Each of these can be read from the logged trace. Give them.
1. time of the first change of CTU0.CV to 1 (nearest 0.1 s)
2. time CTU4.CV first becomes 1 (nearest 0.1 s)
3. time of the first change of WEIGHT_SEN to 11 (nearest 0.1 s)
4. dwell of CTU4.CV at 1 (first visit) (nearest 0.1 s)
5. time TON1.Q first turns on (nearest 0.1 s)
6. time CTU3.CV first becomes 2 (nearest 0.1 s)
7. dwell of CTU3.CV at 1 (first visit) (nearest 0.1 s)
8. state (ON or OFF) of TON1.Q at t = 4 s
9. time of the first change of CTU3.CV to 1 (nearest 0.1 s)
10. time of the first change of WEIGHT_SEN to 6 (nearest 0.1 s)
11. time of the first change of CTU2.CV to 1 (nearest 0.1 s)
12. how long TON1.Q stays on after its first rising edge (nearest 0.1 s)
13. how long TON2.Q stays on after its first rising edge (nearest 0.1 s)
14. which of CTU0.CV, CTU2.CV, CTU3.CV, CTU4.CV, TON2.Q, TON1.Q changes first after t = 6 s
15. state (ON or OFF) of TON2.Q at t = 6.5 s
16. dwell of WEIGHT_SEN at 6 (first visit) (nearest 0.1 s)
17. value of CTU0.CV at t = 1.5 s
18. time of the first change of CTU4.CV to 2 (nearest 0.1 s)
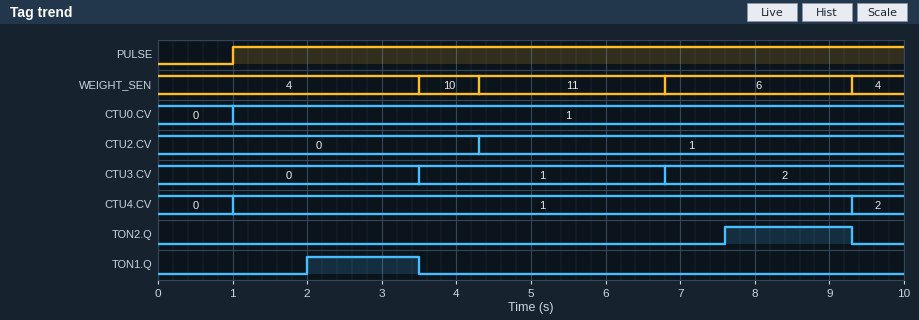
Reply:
1.0 s
1.0 s
4.3 s
8.3 s
2.0 s
6.8 s
3.3 s
OFF
3.5 s
6.8 s
4.3 s
1.5 s
1.7 s
CTU3.CV
OFF
2.5 s
1
9.3 s
